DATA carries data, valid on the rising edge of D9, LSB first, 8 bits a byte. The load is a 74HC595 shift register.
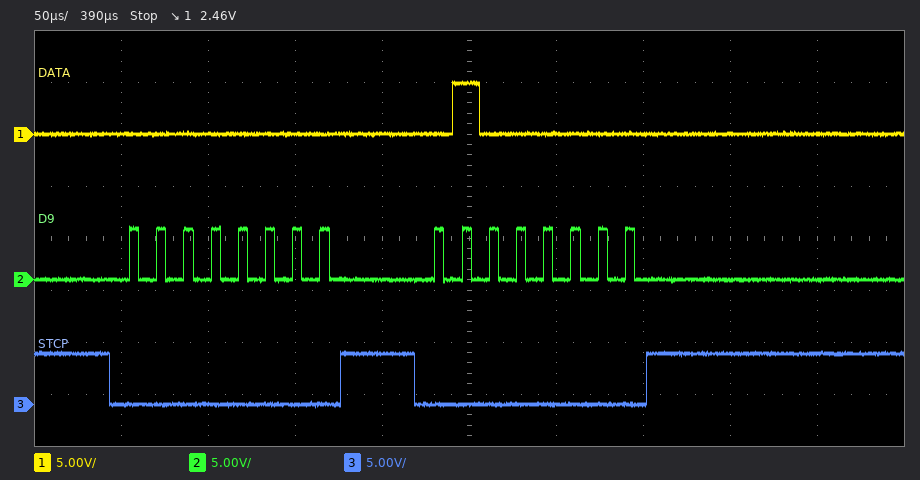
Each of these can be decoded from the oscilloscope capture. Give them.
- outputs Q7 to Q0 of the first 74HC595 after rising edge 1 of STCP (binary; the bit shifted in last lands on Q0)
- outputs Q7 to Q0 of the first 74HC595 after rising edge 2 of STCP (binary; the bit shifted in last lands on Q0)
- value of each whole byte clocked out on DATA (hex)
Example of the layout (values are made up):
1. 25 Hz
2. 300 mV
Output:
1. 00000000
2. 01000000
3. 0x00 0x02
